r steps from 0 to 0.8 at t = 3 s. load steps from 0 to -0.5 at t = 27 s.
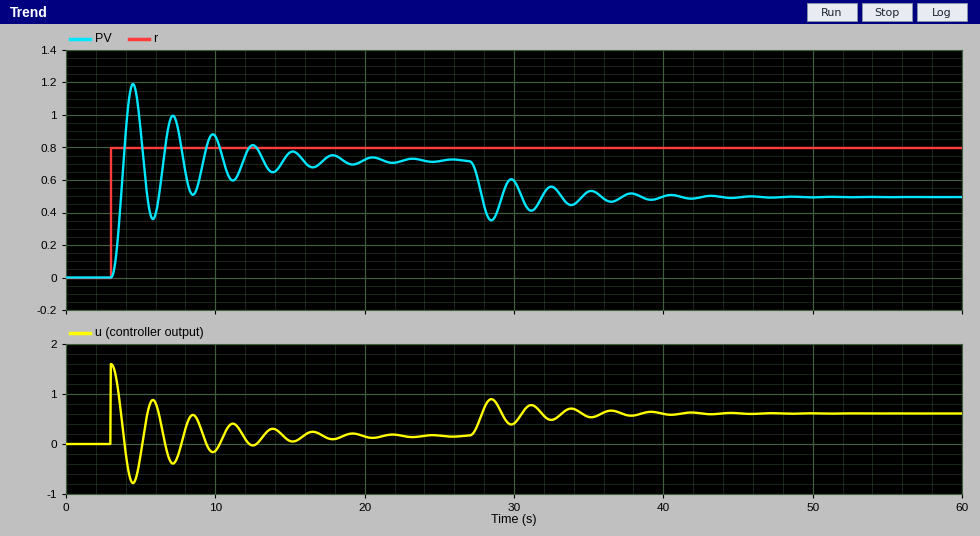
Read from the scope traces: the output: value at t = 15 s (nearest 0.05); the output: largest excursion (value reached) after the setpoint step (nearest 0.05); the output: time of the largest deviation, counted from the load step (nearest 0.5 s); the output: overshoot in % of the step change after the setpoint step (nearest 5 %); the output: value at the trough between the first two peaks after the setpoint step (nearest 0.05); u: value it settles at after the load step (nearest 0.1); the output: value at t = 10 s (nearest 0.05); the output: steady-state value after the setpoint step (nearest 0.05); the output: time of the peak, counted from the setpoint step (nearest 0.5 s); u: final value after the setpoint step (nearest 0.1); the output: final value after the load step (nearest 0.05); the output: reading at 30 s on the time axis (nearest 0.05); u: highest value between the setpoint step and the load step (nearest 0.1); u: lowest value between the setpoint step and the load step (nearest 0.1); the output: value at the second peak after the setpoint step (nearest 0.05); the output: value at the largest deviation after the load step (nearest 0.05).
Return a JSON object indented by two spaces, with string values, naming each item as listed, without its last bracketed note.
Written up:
{
  "the output: value at t = 15 s": "0.75",
  "the output: largest excursion (value reached) after the setpoint step": "1.20",
  "the output: time of the largest deviation, counted from the load step": "1.5 s",
  "the output: overshoot in % of the step change after the setpoint step": "65 %",
  "the output: value at the trough between the first two peaks after the setpoint step": "0.35",
  "u: value it settles at after the load step": "0.6",
  "the output: value at t = 10 s": "0.85",
  "the output: steady-state value after the setpoint step": "0.70",
  "the output: time of the peak, counted from the setpoint step": "1.5 s",
  "u: final value after the setpoint step": "0.2",
  "the output: final value after the load step": "0.50",
  "the output: reading at 30 s on the time axis": "0.60",
  "u: highest value between the setpoint step and the load step": "1.6",
  "u: lowest value between the setpoint step and the load step": "-0.8",
  "the output: value at the second peak after the setpoint step": "1.00",
  "the output: value at the largest deviation after the load step": "0.35"
}
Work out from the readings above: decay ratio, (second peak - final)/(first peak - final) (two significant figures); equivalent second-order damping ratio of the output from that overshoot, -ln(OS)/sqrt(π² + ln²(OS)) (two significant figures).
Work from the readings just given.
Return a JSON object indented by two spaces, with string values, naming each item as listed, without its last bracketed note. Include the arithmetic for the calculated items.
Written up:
{
  "decay ratio, (second peak - final)/(first peak - final)": "(1 - 0.7) / (1.2 - 0.7) = 0.60",
  "equivalent second-order damping ratio of the output from that overshoot, -ln(OS)/sqrt(π² + ln²(OS))": "ln(0.65) = -0.431; 0.431 / sqrt(9.870 + 0.186) = 0.14"
}
